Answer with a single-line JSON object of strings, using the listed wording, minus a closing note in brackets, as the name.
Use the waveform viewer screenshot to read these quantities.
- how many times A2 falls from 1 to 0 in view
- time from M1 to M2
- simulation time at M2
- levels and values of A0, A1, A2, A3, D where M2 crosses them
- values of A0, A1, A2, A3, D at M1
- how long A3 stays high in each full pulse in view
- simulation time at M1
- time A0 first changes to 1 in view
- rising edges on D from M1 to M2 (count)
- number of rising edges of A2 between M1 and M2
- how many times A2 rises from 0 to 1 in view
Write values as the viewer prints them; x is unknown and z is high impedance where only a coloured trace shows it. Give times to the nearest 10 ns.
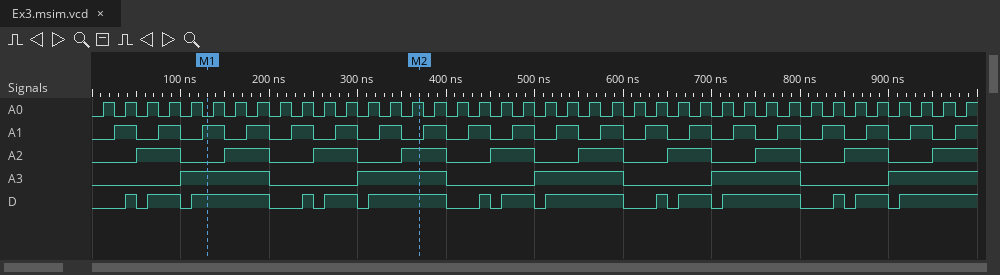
{"how many times A2 falls from 1 to 0 in view": "9", "time from M1 to M2": "240 ns", "simulation time at M2": "370 ns", "levels and values of A0, A1, A2, A3, D where M2 crosses them": "A0=1, A1=0, A2=1, A3=1, D=1", "values of A0, A1, A2, A3, D at M1": "A0=0, A1=1, A2=0, A3=1, D=1", "how long A3 stays high in each full pulse in view": "100 ns, 100 ns, 100 ns, 100 ns", "simulation time at M1": "130 ns", "time A0 first changes to 1 in view": "10 ns", "rising edges on D from M1 to M2": "3", "number of rising edges of A2 between M1 and M2": "3", "how many times A2 rises from 0 to 1 in view": "10"}
